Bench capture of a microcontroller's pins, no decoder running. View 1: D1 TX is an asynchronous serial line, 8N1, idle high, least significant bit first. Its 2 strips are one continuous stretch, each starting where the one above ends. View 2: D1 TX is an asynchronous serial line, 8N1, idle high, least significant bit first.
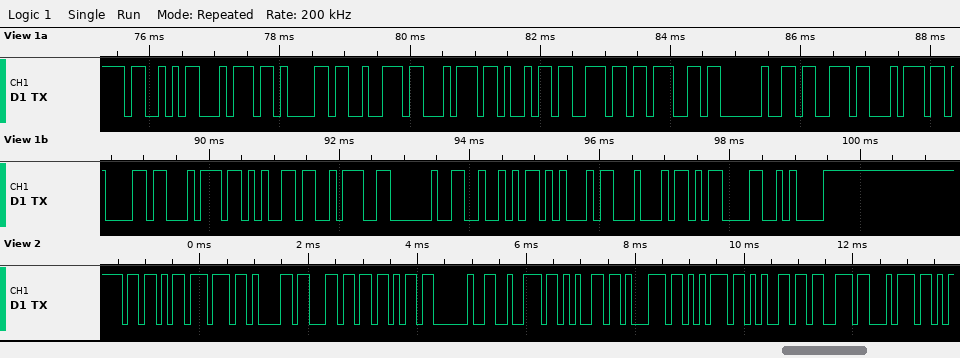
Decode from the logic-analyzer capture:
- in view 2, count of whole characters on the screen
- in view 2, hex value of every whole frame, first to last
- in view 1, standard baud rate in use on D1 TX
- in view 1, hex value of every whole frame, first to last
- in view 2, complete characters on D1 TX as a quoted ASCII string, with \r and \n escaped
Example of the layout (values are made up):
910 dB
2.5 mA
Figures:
13
5B 77 61 6C 6B 20 72 65 71 75 65 73 74
9600 baud
53 74 61 72 74 69 6E 67 20 73 74 61 74 65 3A 20 52 45 44 0D 0A
"[walk request"
